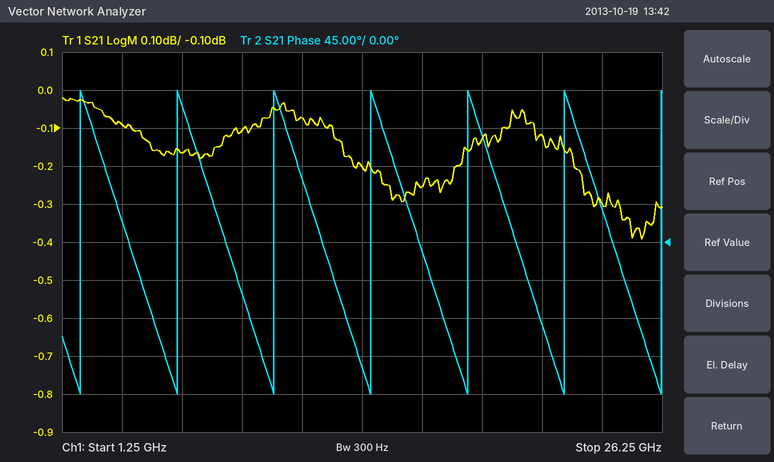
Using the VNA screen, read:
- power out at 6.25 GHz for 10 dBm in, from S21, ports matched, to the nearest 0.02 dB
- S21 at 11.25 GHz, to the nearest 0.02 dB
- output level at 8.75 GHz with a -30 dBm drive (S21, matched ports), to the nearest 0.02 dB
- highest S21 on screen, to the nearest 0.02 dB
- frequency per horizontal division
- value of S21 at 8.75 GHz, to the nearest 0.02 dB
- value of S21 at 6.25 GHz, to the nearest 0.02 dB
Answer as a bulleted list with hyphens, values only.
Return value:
- 9.84 dBm
- -0.08 dB
- -30.10 dBm
- -0.02 dB
- 2.5 GHz
- -0.10 dB
- -0.16 dB
